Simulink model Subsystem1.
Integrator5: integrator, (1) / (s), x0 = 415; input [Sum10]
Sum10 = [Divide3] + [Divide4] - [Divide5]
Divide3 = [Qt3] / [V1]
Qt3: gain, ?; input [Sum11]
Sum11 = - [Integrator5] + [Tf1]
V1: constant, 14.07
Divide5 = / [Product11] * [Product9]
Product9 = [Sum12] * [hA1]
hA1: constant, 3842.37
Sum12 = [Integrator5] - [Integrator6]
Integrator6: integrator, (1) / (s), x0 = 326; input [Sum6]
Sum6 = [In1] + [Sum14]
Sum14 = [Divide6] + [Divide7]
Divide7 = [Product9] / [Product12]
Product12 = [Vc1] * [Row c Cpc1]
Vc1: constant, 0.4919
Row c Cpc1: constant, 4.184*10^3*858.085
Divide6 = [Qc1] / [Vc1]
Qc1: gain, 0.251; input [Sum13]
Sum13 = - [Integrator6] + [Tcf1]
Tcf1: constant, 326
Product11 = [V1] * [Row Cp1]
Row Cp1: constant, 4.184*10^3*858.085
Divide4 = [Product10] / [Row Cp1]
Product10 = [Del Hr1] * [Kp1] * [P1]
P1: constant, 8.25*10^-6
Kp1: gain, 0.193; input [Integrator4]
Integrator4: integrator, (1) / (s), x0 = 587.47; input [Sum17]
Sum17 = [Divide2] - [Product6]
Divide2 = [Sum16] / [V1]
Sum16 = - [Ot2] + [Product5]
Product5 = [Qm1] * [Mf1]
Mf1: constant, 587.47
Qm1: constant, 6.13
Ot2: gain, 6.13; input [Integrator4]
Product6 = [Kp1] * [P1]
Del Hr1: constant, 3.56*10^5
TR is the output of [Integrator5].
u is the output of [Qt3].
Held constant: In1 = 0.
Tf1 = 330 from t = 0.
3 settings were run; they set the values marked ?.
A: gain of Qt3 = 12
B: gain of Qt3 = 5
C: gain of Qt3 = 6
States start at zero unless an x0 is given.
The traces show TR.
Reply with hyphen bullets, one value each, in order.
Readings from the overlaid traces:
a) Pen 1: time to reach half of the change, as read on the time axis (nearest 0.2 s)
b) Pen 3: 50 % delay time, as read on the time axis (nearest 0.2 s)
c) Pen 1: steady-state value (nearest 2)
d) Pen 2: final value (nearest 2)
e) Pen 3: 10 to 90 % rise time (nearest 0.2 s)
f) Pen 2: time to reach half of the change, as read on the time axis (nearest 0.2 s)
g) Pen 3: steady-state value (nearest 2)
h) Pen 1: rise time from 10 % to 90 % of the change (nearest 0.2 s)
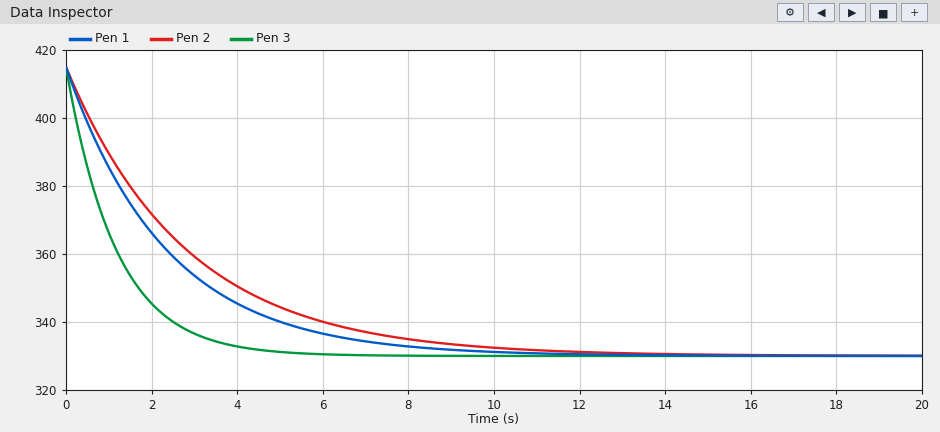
- 1.6 s
- 0.8 s
- 330
- 330
- 2.6 s
- 2.0 s
- 330
- 5.2 s
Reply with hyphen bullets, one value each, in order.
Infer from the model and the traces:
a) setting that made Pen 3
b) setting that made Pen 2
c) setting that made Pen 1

- A
- B
- C
